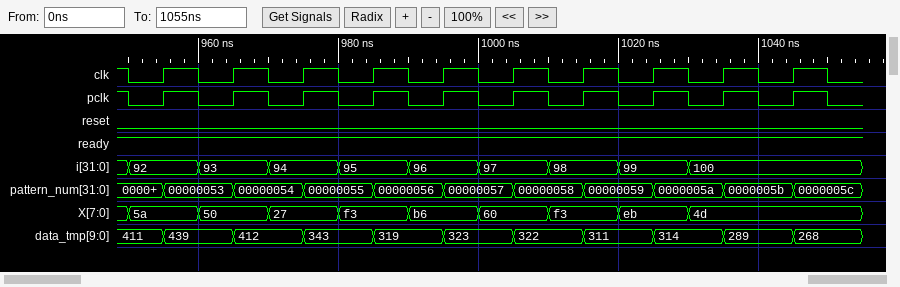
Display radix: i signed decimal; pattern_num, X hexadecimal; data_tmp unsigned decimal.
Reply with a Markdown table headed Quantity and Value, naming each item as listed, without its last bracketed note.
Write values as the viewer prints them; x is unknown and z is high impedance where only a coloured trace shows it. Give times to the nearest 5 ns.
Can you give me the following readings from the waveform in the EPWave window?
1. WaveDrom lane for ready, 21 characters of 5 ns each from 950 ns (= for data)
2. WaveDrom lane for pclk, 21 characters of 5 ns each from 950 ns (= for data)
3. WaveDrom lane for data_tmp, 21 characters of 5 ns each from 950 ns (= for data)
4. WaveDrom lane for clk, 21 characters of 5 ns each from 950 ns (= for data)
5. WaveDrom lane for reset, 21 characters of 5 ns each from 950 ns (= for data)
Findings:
| Quantity | Value |
|---|---|
| WaveDrom lane for ready, 21 characters of 5 ns each from 950 ns | {name: 'ready', wave: '1....................'} |
| WaveDrom lane for pclk, 21 characters of 5 ns each from 950 ns | {name: 'pclk', wave: '010101010101010101010'} |
| WaveDrom lane for data_tmp, 21 characters of 5 ns each from 950 ns | {name: 'data_tmp', wave: '==.=.=.=.=.=.=.=.=.=.', data: '411 439 412 343 319 323 322 311 314 289 268'} |
| WaveDrom lane for clk, 21 characters of 5 ns each from 950 ns | {name: 'clk', wave: '010101010101010101010'} |
| WaveDrom lane for reset, 21 characters of 5 ns each from 950 ns | {name: 'reset', wave: '0....................'} |
